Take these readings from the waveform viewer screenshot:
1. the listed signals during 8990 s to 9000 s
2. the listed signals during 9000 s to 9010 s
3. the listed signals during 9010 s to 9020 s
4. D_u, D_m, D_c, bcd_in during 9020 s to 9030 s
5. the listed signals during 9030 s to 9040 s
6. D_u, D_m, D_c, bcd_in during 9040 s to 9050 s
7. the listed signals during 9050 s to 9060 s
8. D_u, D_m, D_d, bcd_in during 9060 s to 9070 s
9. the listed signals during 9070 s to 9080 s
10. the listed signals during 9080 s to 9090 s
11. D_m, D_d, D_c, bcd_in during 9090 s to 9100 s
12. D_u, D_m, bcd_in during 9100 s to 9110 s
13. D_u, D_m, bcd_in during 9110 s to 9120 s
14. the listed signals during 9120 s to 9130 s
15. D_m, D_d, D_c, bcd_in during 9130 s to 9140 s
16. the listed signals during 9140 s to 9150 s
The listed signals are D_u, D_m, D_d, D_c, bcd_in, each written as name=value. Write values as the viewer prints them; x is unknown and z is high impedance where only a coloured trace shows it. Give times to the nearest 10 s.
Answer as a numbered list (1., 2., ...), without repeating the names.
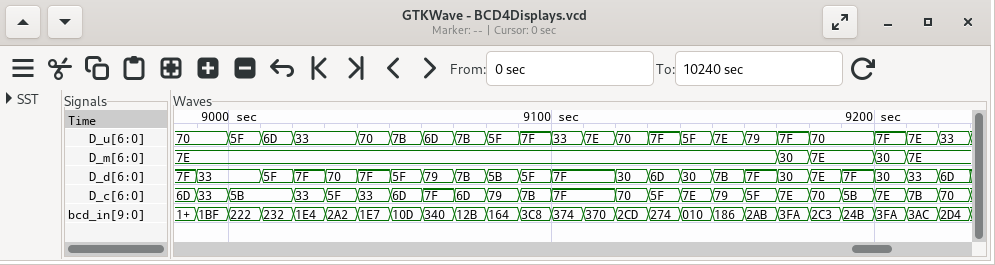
1. D_u=70, D_m=7E, D_d=33, D_c=33, bcd_in=1BF
2. D_u=5F, D_m=7E, D_d=33, D_c=5B, bcd_in=222
3. D_u=6D, D_m=7E, D_d=5F, D_c=5B, bcd_in=232
4. D_u=33, D_m=7E, D_c=33, bcd_in=1E4
5. D_u=33, D_m=7E, D_d=70, D_c=5F, bcd_in=2A2
6. D_u=70, D_m=7E, D_c=33, bcd_in=1E7
7. D_u=7B, D_m=7E, D_d=5F, D_c=6D, bcd_in=10D
8. D_u=6D, D_m=7E, D_d=79, bcd_in=340
9. D_u=7B, D_m=7E, D_d=7B, D_c=6D, bcd_in=12B
10. D_u=5F, D_m=7E, D_d=5B, D_c=79, bcd_in=164
11. D_m=7E, D_d=5F, D_c=7B, bcd_in=3C8
12. D_u=33, D_m=7E, bcd_in=374
13. D_u=7E, D_m=7E, bcd_in=370
14. D_u=70, D_m=7E, D_d=30, D_c=70, bcd_in=2CD
15. D_m=7E, D_d=6D, D_c=5F, bcd_in=274
16. D_u=5F, D_m=7E, D_d=30, D_c=7E, bcd_in=010
